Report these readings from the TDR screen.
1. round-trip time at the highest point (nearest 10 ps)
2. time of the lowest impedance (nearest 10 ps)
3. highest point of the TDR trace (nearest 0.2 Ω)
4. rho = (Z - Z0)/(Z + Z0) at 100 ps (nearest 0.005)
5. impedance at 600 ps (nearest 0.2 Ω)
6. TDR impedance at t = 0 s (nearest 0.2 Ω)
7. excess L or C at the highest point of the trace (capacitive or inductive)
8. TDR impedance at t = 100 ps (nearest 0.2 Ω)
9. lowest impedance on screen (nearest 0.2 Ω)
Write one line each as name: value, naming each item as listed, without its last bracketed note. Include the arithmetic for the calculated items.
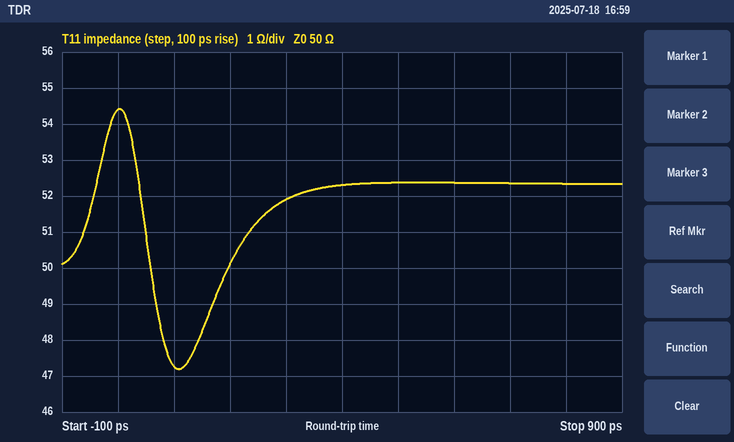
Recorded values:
round-trip time at the highest point: 0 ps
time of the lowest impedance: 110 ps
highest point of the TDR trace: 54.4 Ω
rho = (Z - Z0)/(Z + Z0) at 100 ps: (47.2 − 50)/(47.2 + 50) ≈ -0.0288, so -0.030 to the nearest 0.005
impedance at 600 ps: 52.4 Ω
TDR impedance at t = 0 s: 54.4 Ω
excess L or C at the highest point of the trace: inductive
TDR impedance at t = 100 ps: 47.2 Ω
lowest impedance on screen: 47.2 Ω
